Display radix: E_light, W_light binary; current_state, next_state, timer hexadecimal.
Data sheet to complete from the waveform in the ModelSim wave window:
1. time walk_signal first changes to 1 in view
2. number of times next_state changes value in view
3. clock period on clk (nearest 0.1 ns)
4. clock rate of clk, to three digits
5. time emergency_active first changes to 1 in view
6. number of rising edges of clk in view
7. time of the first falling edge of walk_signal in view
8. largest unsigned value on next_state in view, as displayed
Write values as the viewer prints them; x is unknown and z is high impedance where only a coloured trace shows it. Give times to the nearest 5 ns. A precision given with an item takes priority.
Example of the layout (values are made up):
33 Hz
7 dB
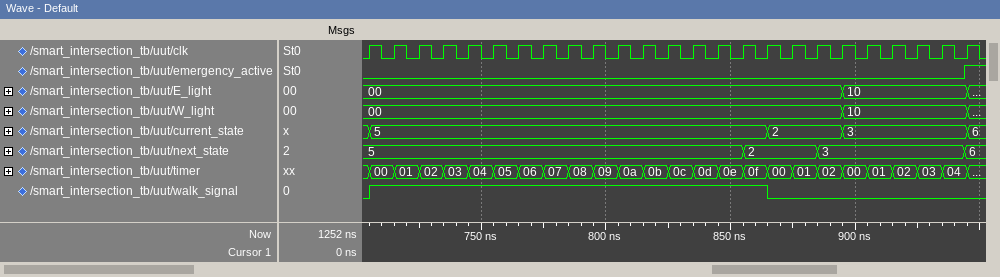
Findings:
705 ns
3
10 ns
100 MHz
945 ns
25
865 ns
6
